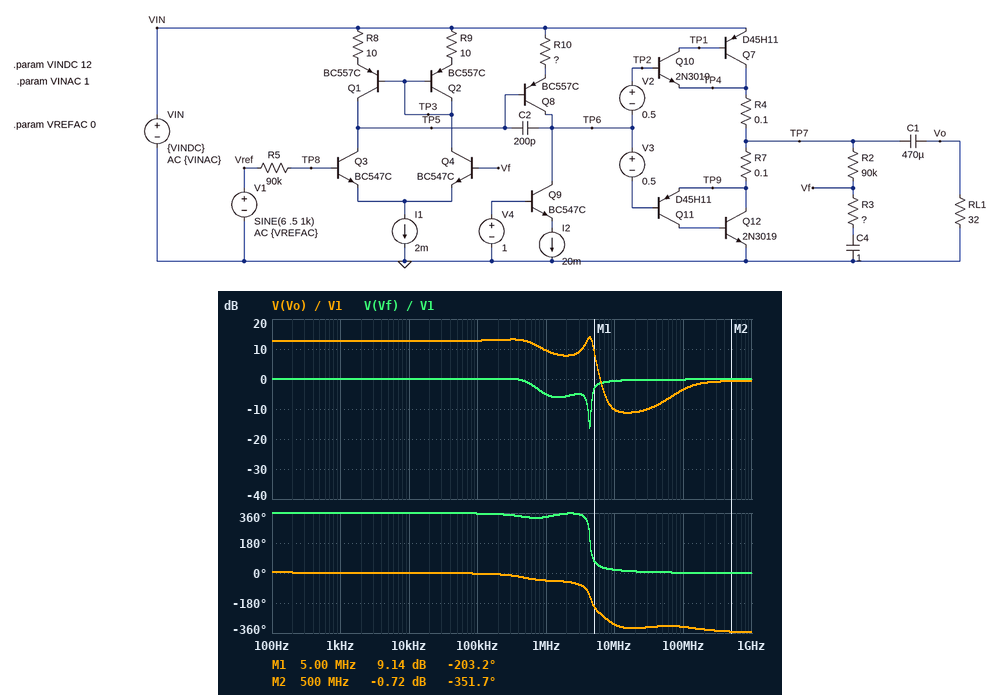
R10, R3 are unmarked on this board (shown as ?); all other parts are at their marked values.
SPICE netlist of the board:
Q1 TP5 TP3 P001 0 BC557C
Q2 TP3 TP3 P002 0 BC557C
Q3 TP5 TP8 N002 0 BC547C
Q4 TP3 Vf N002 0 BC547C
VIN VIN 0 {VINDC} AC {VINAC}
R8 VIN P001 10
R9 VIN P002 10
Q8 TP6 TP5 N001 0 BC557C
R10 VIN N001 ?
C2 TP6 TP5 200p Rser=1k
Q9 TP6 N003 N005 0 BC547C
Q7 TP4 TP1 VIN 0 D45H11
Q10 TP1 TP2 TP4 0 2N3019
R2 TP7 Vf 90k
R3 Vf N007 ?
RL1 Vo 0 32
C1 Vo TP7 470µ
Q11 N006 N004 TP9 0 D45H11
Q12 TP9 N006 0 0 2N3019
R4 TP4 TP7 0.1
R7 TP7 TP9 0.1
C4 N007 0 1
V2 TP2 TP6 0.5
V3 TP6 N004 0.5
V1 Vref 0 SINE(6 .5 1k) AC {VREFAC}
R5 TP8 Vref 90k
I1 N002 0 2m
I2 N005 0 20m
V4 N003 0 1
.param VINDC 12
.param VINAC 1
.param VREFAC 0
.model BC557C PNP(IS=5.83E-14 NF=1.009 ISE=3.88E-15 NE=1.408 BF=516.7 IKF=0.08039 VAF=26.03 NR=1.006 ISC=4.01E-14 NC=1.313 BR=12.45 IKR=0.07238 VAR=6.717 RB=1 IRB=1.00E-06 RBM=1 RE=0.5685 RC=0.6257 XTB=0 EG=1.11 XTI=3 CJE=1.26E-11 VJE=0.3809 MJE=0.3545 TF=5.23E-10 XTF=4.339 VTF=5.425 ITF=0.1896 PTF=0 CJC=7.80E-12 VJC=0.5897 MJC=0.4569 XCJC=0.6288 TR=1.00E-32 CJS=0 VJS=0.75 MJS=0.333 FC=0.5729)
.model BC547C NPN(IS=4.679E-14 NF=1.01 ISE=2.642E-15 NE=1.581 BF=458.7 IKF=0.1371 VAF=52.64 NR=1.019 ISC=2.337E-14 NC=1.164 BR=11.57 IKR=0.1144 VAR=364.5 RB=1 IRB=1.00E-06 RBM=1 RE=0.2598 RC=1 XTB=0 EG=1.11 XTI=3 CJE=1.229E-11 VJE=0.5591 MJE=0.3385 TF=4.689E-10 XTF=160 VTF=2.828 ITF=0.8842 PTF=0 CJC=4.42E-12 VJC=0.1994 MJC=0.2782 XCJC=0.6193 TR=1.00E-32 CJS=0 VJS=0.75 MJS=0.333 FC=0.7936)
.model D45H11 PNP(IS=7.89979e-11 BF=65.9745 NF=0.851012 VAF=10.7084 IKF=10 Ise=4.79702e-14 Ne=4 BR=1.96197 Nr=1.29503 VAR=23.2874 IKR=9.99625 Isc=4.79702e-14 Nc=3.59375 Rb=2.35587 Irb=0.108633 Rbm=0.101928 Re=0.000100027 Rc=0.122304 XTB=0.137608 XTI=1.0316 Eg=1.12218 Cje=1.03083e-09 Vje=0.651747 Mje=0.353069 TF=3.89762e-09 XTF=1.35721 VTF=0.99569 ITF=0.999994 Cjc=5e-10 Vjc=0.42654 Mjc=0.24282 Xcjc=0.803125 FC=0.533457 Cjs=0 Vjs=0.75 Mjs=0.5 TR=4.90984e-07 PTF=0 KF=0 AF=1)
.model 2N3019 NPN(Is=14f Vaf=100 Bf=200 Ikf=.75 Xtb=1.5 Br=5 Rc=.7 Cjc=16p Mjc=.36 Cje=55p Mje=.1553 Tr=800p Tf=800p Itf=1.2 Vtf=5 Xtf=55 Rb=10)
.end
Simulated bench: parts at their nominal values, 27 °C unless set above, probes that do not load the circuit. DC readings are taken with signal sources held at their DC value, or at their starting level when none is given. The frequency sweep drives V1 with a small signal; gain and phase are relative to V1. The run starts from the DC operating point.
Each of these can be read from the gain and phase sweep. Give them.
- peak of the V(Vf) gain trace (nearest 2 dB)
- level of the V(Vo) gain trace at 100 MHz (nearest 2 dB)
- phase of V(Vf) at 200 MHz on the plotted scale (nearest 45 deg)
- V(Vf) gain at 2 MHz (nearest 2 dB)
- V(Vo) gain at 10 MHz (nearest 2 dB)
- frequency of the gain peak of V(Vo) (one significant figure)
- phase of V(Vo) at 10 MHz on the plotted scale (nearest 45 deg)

0 dB
-4 dB
0 deg
-6 dB
-10 dB
4 MHz
-315 deg
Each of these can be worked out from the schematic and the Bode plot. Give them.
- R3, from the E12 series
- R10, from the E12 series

27 kΩ
18 Ω
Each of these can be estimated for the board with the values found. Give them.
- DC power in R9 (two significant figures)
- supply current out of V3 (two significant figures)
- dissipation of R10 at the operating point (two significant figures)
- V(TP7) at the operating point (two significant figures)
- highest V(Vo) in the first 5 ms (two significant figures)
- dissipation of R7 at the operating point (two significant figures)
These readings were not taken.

9.4 µW
5.3 µA
7.2 mW
6.0 V
2.1 V
900 µW
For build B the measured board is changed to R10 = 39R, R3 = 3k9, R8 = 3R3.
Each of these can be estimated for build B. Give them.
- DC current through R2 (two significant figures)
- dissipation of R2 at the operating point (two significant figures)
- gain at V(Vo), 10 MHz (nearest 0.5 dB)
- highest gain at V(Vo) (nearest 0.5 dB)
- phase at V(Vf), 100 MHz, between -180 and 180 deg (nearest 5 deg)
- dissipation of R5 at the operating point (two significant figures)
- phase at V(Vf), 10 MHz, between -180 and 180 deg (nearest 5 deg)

1.7 µA
270 nW
-10.0 dB
27.5 dB
10 deg
470 nW
70 deg
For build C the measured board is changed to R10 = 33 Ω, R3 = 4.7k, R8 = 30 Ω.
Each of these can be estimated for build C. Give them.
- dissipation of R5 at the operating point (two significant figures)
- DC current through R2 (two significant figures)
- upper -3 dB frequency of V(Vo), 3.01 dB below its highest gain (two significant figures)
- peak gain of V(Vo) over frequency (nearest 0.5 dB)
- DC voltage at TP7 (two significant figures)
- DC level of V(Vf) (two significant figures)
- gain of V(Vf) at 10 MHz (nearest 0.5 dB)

250 nW
2.3 µA
240 kHz
26.0 dB
6.1 V
5.9 V
-5.0 dB
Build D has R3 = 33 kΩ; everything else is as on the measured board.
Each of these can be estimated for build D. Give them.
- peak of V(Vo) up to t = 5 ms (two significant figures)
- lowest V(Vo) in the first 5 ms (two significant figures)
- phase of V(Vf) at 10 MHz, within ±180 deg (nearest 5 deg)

1.8 V
-1.9 V
15 deg
